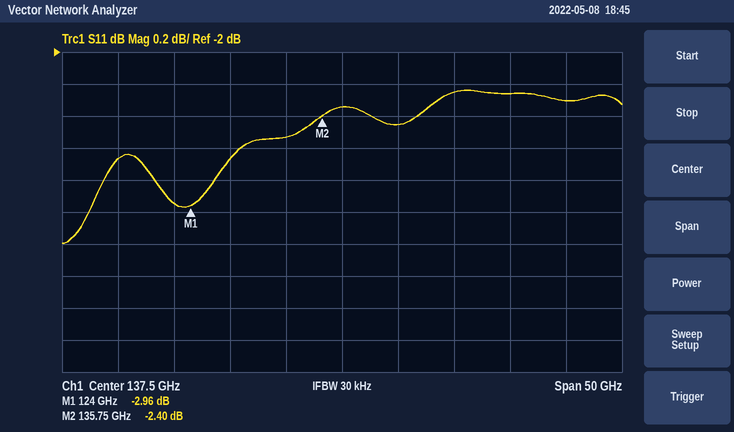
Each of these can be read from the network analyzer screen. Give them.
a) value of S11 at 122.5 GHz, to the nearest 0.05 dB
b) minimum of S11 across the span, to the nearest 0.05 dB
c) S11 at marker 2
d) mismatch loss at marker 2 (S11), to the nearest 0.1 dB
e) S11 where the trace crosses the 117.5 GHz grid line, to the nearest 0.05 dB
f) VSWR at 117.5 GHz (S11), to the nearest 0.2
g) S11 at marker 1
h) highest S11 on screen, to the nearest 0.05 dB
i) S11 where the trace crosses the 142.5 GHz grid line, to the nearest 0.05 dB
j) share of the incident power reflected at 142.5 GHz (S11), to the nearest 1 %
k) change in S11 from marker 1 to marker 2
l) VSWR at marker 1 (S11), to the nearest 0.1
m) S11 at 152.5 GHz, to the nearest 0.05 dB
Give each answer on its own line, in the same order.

-2.95 dB
-3.20 dB
-2.40 dB
3.7 dB
-2.65 dB
6.6
-2.96 dB
-2.25 dB
-2.45 dB
57 %
0.56 dB
5.9
-2.25 dB
